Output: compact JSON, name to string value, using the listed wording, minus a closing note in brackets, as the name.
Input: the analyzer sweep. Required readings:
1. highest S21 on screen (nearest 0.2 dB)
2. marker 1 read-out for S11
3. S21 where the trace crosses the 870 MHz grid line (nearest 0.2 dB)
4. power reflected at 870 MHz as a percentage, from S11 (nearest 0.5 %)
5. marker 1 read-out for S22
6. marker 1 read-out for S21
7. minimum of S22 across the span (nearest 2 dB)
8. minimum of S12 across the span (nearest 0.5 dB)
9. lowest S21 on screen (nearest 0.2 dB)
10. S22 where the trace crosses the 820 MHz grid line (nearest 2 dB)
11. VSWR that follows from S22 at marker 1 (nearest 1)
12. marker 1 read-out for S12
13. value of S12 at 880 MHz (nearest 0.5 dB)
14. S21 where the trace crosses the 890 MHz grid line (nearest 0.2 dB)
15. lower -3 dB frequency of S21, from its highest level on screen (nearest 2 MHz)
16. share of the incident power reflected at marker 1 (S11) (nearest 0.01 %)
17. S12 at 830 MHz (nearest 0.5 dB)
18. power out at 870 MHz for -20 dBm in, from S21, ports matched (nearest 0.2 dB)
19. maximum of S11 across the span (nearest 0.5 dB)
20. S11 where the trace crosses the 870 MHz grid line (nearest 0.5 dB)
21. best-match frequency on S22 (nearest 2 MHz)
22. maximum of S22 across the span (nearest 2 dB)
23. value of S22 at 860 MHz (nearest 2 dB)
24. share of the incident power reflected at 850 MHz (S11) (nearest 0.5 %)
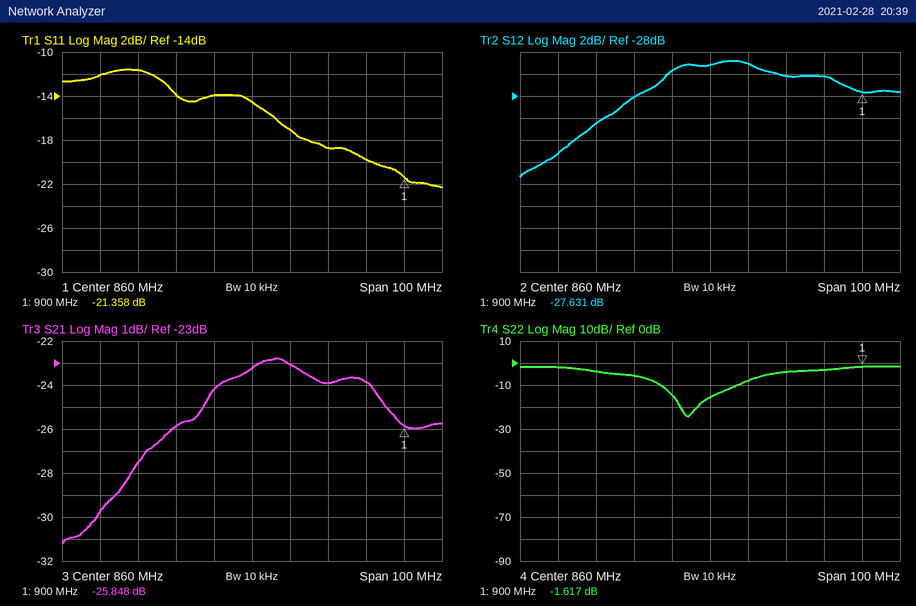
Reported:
{"highest S21 on screen": "-22.8 dB", "marker 1 read-out for S11": "-21.358 dB", "S21 where the trace crosses the 870 MHz grid line": "-23.0 dB", "power reflected at 870 MHz as a percentage, from S11": "2.0 %", "marker 1 read-out for S22": "-1.617 dB", "marker 1 read-out for S21": "-25.848 dB", "minimum of S22 across the span": "-24 dB", "minimum of S12 across the span": "-35.5 dB", "lowest S21 on screen": "-31.2 dB", "S22 where the trace crosses the 820 MHz grid line": "-2 dB", "VSWR that follows from S22 at marker 1": "11", "marker 1 read-out for S12": "-27.631 dB", "value of S12 at 880 MHz": "-26.0 dB", "S21 where the trace crosses the 890 MHz grid line": "-23.8 dB", "lower -3 dB frequency of S21, from its highest level on screen": "840 MHz", "share of the incident power reflected at marker 1 (S11)": "0.73 %", "S12 at 830 MHz": "-30.5 dB", "power out at 870 MHz for -20 dBm in, from S21, ports matched": "-43.0 dBm", "maximum of S11 across the span": "-11.5 dB", "S11 where the trace crosses the 870 MHz grid line": "-17.0 dB", "best-match frequency on S22": "854 MHz", "maximum of S22 across the span": "-2 dB", "value of S22 at 860 MHz": "-16 dB", "share of the incident power reflected at 850 MHz (S11)": "4.0 %"}
